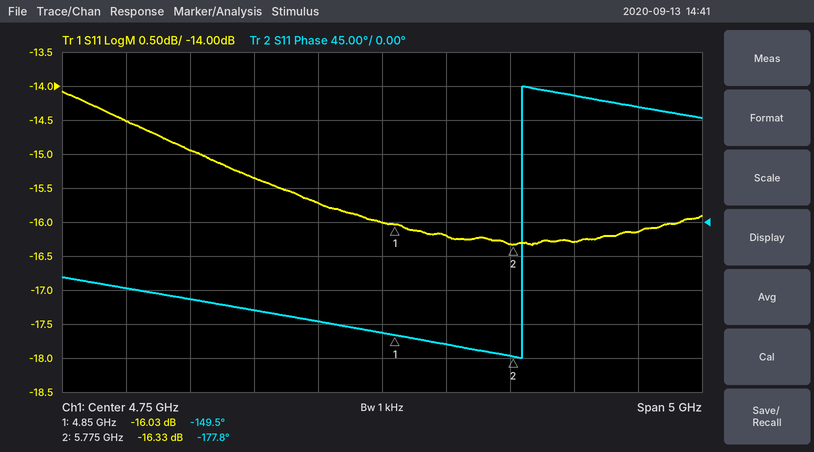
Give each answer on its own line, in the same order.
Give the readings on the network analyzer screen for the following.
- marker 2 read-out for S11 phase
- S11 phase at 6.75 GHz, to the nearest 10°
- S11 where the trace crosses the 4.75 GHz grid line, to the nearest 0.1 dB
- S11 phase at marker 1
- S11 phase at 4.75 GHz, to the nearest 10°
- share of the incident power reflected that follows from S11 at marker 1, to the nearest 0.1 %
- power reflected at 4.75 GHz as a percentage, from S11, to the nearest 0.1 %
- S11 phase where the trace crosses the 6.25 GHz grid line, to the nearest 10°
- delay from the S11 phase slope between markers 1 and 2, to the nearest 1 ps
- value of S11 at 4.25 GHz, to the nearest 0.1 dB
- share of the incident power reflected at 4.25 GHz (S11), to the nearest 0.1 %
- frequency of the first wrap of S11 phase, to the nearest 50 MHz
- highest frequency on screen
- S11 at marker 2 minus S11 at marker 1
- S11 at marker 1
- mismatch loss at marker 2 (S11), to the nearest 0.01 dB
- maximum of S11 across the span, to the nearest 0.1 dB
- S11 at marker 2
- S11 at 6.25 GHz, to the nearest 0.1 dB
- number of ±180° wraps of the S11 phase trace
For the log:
-177.8°
150°
-16.0 dB
-149.5°
-150°
2.5 %
2.5 %
170°
85 ps
-15.7 dB
2.7 %
5.85 GHz
7.25 GHz
-0.30 dB
-16.03 dB
0.10 dB
-14.1 dB
-16.33 dB
-16.3 dB
1
